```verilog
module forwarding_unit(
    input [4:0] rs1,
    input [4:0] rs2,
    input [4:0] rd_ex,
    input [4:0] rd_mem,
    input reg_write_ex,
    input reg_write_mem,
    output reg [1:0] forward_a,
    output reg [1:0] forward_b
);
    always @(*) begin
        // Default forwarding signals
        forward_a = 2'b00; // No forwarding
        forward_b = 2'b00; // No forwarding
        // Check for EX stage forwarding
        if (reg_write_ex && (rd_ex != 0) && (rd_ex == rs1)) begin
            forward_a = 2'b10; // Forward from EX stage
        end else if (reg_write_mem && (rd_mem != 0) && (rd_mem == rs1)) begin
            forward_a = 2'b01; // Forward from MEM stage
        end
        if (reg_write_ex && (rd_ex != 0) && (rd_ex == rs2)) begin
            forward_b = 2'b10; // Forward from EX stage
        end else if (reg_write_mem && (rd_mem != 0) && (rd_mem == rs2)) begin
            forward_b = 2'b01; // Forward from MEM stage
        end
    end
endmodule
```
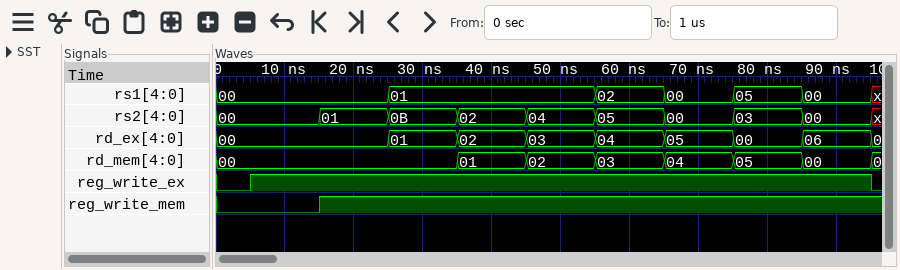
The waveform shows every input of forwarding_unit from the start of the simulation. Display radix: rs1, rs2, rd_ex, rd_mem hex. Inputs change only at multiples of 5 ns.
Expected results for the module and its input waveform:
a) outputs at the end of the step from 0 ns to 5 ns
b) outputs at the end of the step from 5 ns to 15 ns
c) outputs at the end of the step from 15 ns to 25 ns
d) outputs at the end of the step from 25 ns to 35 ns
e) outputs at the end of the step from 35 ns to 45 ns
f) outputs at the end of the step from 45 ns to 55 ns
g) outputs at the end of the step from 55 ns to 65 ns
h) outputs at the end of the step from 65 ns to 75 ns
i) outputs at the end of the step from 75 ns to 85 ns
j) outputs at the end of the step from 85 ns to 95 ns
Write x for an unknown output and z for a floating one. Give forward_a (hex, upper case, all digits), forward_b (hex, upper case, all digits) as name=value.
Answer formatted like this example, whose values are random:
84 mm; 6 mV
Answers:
forward_a=0, forward_b=0; forward_a=0, forward_b=0; forward_a=0, forward_b=0; forward_a=2, forward_b=0; forward_a=1, forward_b=2; forward_a=0, forward_b=0; forward_a=0, forward_b=0; forward_a=0, forward_b=0; forward_a=1, forward_b=0; forward_a=0, forward_b=0
